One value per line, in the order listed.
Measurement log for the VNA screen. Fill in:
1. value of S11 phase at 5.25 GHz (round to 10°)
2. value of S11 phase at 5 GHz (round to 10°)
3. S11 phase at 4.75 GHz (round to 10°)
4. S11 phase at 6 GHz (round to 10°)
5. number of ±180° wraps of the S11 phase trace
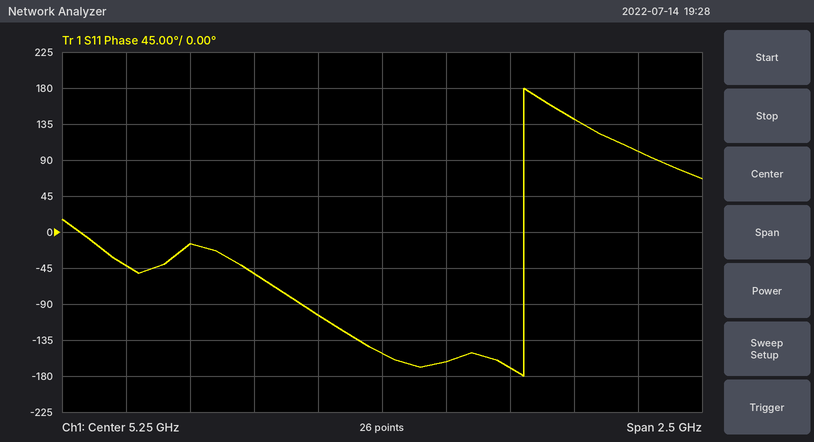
-150°
-100°
-50°
140°
1
